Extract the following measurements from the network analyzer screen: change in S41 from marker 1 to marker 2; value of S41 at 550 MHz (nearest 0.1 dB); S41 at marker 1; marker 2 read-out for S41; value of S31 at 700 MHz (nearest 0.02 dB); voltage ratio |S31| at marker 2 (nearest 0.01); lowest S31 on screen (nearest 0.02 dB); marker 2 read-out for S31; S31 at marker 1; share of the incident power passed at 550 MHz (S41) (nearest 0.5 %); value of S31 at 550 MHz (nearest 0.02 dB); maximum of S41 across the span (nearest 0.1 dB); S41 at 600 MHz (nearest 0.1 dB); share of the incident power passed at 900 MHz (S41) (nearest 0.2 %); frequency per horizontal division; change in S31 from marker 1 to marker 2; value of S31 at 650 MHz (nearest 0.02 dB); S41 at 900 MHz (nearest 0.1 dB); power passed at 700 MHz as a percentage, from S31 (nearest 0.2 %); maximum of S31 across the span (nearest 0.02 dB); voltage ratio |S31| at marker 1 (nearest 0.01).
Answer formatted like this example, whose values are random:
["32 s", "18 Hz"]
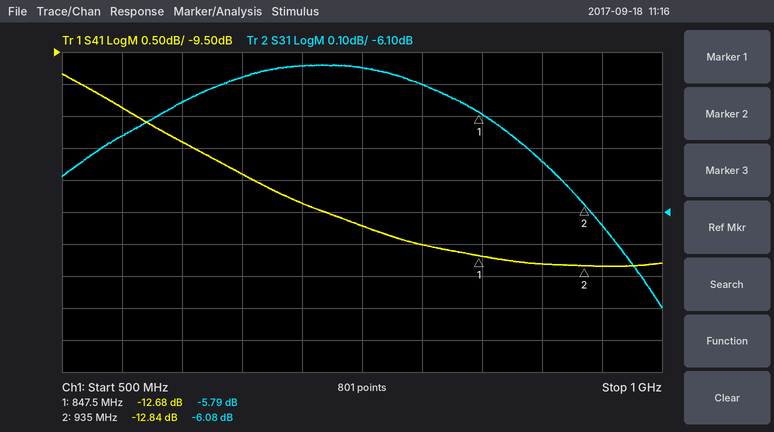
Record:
["-0.16 dB", "-10.4 dB", "-12.68 dB", "-12.84 dB", "-5.64 dB", "0.50", "-6.40 dB", "-6.08 dB", "-5.79 dB", "9.0 %", "-5.86 dB", "-9.8 dB", "-10.9 dB", "5.2 %", "50 MHz", "-0.29 dB", "-5.68 dB", "-12.8 dB", "27.2 %", "-5.64 dB", "0.51"]
